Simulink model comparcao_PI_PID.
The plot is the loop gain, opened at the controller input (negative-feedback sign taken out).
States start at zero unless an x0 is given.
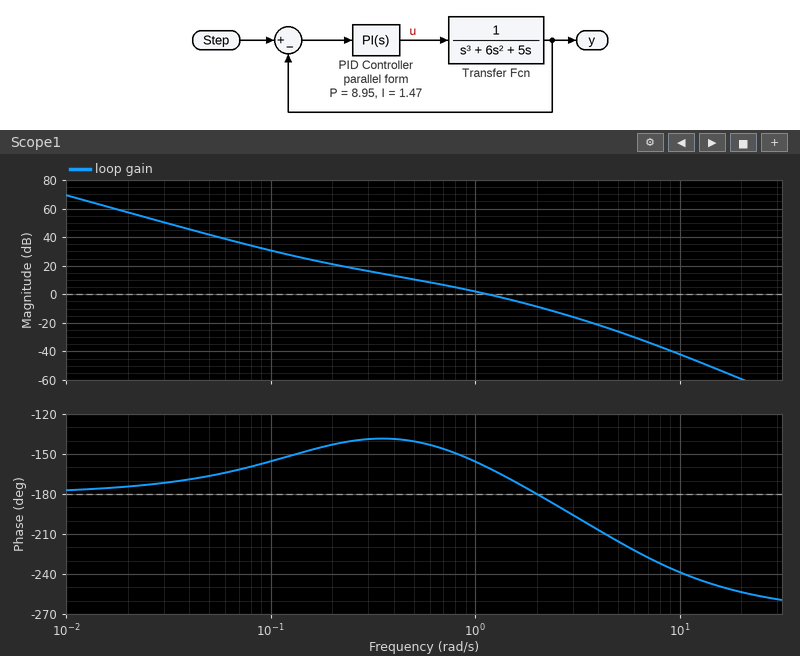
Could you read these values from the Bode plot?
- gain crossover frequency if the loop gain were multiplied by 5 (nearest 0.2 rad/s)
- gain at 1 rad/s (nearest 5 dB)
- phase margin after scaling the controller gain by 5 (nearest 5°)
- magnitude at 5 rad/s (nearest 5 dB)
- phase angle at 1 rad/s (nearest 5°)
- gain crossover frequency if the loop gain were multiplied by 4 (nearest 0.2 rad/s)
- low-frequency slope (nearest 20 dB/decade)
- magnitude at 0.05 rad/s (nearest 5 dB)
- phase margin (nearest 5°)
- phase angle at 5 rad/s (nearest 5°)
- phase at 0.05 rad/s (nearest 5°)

2.8 rad/s
0 dB
-10°
-25 dB
-155°
2.4 rad/s
-40 dB/decade
40 dB
20°
-215°
-165°
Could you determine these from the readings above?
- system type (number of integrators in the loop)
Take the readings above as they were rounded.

2
